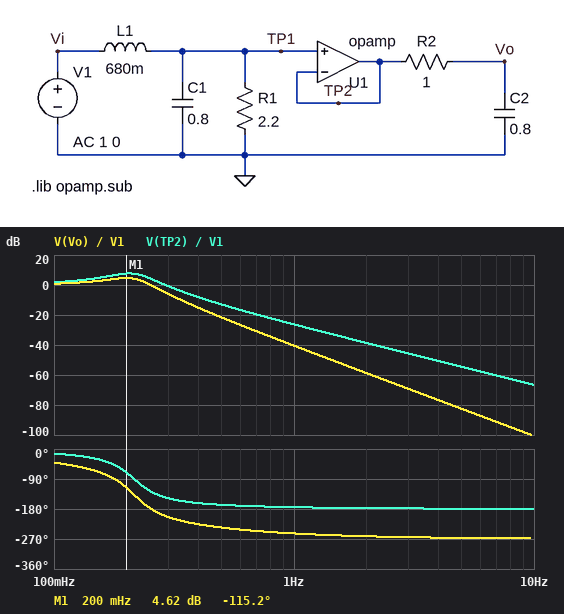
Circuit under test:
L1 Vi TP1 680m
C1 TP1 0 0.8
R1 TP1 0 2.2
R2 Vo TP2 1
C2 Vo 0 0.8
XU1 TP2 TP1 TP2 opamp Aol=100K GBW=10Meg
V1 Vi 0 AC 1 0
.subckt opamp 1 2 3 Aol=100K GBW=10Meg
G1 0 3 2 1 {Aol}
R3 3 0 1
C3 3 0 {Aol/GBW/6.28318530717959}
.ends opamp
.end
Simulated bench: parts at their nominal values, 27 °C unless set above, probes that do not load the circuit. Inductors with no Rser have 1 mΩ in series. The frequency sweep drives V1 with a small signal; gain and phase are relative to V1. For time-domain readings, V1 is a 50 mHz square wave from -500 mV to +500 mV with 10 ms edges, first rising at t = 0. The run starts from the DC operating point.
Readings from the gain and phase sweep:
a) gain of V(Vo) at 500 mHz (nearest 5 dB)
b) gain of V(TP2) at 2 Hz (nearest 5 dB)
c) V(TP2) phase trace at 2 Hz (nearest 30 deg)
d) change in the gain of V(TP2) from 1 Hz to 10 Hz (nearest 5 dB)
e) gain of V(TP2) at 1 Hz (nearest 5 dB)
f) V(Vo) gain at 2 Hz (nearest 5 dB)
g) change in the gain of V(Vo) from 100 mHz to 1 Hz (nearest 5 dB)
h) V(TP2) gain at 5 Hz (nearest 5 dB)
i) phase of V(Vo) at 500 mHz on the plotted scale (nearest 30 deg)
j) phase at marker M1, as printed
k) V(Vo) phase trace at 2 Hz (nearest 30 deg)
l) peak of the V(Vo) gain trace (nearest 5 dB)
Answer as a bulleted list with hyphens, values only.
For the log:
- -20 dB
- -40 dB
- -180 deg
- -40 dB
- -25 dB
- -60 dB
- -40 dB
- -55 dB
- -240 deg
- -115.2 deg
- -270 deg
- 5 dB
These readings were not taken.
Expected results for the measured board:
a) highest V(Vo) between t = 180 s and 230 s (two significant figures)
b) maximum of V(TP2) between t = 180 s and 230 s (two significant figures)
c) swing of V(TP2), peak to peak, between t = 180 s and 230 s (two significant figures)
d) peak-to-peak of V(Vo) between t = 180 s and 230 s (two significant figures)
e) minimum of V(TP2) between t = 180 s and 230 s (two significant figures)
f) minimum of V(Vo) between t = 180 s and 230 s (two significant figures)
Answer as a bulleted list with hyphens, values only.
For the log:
- 790 mV
- 980 mV
- 2.0 V
- 1.6 V
- -980 mV
- -790 mV
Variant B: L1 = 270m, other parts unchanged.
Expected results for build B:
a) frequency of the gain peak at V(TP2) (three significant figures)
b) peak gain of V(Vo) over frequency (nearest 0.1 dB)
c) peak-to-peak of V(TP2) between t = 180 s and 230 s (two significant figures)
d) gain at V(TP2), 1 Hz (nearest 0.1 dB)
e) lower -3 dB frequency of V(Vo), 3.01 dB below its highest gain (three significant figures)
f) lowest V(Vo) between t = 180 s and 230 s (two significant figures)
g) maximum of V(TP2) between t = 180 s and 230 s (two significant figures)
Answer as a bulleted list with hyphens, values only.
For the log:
- 336 mHz
- 5.8 dB
- 2.4 V
- -17.6 dB
- 270 mHz
- -750 mV
- 1.2 V
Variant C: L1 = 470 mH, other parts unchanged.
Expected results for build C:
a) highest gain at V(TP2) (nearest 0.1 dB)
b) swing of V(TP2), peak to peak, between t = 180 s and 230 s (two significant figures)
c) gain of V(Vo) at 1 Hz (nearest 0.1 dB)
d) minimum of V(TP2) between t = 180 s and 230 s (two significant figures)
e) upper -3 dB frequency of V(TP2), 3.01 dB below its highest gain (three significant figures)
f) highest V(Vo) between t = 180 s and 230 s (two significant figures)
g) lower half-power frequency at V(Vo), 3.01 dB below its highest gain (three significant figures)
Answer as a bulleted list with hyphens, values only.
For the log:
- 9.3 dB
- 2.2 V
- -37.1 dB
- -1.1 V
- 294 mHz
- 810 mV
- 178 mHz
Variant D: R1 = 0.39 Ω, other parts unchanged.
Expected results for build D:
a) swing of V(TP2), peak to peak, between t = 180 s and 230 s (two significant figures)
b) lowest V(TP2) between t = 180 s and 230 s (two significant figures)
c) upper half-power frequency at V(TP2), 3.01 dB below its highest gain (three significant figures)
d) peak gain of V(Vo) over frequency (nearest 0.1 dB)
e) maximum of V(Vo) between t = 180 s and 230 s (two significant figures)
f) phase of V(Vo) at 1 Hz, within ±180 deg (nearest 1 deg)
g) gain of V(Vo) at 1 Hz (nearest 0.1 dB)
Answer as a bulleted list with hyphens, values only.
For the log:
- 1.0 V
- -500 mV
- 110 mHz
- 0 dB
- 500 mV
- 129 deg
- -41.5 dB
